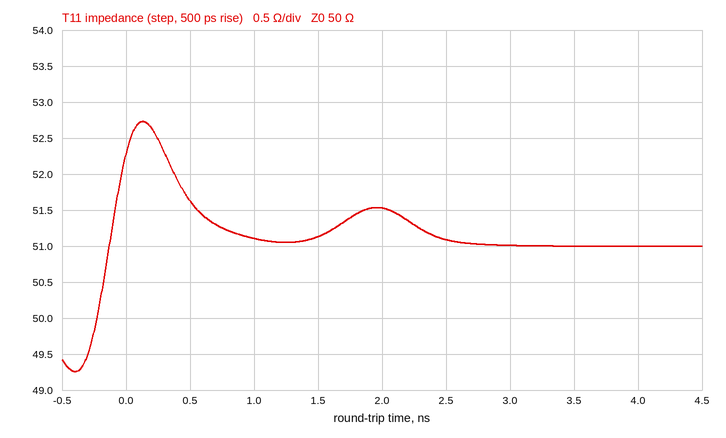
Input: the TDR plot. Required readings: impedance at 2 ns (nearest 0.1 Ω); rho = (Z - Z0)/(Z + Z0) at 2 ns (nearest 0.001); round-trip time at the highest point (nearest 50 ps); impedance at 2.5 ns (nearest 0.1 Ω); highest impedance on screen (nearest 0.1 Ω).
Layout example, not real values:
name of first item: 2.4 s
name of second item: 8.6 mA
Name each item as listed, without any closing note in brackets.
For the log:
impedance at 2 ns: 51.5 Ω
rho = (Z - Z0)/(Z + Z0) at 2 ns: +0.015
round-trip time at the highest point: 150 ps
impedance at 2.5 ns: 51.1 Ω
highest impedance on screen: 52.7 Ω
